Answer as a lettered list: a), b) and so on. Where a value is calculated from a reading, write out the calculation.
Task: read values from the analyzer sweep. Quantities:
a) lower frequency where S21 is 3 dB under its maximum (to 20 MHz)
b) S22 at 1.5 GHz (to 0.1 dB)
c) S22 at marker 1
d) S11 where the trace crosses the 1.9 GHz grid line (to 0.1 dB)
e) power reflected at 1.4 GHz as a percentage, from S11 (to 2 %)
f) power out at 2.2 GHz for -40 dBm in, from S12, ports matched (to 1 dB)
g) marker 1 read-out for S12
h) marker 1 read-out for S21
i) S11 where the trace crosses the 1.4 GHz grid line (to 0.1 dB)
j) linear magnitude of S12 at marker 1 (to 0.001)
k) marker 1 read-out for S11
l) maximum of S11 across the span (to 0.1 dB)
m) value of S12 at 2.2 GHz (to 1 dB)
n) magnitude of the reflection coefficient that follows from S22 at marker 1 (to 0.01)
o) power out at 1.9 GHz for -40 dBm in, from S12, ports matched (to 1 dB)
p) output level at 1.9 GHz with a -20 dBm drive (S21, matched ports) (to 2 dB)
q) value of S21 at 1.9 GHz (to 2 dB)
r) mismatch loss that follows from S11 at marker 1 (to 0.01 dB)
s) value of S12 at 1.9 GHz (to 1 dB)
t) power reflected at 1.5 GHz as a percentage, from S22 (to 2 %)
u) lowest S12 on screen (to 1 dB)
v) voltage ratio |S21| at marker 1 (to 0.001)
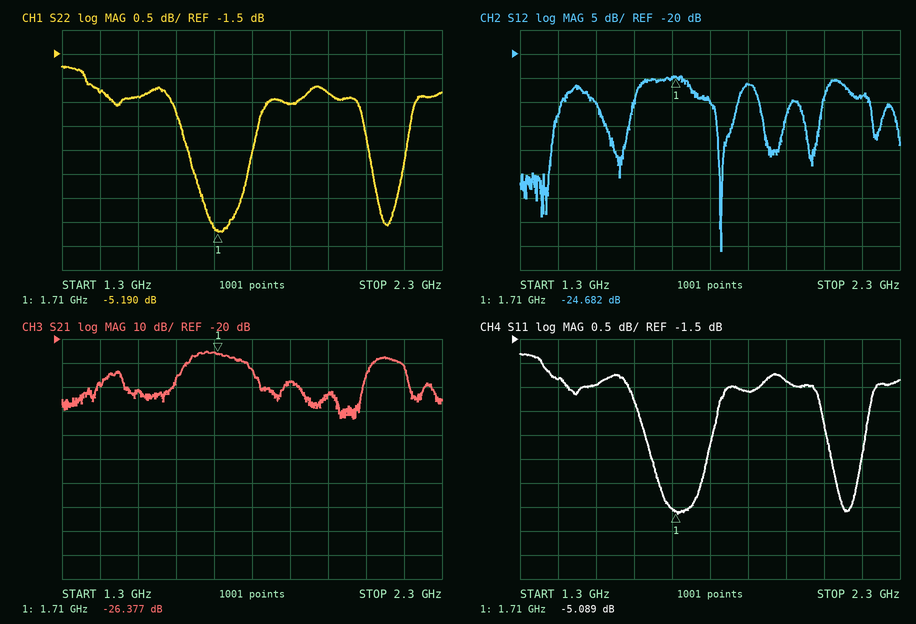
a) 1.64 GHz
b) -2.4 dB
c) -5.190 dB
d) -2.6 dB
e) 10^(-2.3/10) ≈ 58.9 %, so 58 % to the nearest 2 %
f) -40 dBm + (-29 dB) = -69 dBm
g) -24.682 dB
h) -26.377 dB
i) -2.3 dB
j) 10^(-24.682/20) ≈ 0.058
k) -5.089 dB
l) -1.8 dB
m) -29 dB
n) 10^(-5.19/20) ≈ 0.55
o) -40 dBm + (-26 dB) = -66 dBm
p) -20 dBm + (-38 dB) = -58 dBm
q) -38 dB
r) −10 log10(1 − 10^(-5.089/10)) ≈ 1.61 dB
s) -26 dB
t) 10^(-2.4/10) ≈ 58 %
u) -61 dB
v) 10^(-26.377/20) ≈ 0.048
